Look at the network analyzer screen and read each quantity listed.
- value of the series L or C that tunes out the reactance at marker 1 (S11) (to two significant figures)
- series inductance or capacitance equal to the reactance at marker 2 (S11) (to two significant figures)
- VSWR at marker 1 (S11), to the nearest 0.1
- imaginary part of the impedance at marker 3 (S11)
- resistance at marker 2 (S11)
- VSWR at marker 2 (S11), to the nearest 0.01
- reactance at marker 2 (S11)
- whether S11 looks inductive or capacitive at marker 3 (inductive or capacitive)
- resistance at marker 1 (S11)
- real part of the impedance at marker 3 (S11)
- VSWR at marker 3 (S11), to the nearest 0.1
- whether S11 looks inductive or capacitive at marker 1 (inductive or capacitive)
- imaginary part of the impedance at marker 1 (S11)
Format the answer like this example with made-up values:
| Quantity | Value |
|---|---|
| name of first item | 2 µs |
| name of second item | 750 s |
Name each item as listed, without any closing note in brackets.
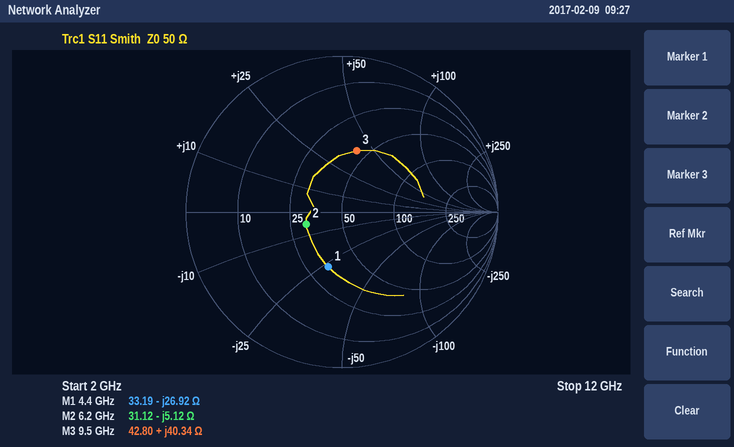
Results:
| Quantity | Value |
|---|---|
| value of the series L or C that tunes out the reactance at marker 1 (S11) | 970 pH |
| series inductance or capacitance equal to the reactance at marker 2 (S11) | 5.0 pF |
| VSWR at marker 1 (S11), to the nearest 0.1 | 2.1 |
| imaginary part of the impedance at marker 3 | +40.34 Ω |
| resistance at marker 2 | 31.12 Ω |
| VSWR at marker 2 (S11), to the nearest 0.01 | 1.63 |
| reactance at marker 2 | -5.12 Ω |
| whether S11 looks inductive or capacitive at marker 3 | inductive |
| resistance at marker 1 | 33.19 Ω |
| real part of the impedance at marker 3 | 42.80 Ω |
| VSWR at marker 3 (S11), to the nearest 0.1 | 2.4 |
| whether S11 looks inductive or capacitive at marker 1 | capacitive |
| imaginary part of the impedance at marker 1 | -26.92 Ω |
